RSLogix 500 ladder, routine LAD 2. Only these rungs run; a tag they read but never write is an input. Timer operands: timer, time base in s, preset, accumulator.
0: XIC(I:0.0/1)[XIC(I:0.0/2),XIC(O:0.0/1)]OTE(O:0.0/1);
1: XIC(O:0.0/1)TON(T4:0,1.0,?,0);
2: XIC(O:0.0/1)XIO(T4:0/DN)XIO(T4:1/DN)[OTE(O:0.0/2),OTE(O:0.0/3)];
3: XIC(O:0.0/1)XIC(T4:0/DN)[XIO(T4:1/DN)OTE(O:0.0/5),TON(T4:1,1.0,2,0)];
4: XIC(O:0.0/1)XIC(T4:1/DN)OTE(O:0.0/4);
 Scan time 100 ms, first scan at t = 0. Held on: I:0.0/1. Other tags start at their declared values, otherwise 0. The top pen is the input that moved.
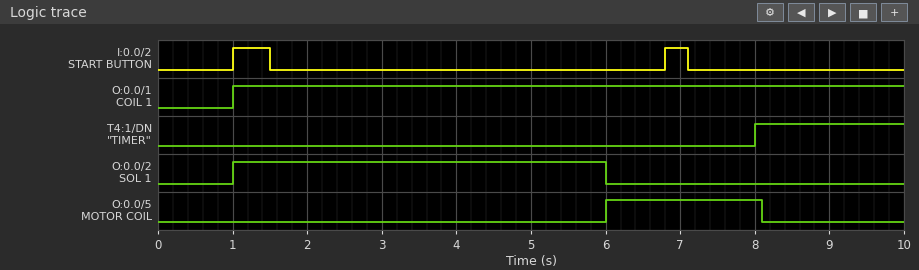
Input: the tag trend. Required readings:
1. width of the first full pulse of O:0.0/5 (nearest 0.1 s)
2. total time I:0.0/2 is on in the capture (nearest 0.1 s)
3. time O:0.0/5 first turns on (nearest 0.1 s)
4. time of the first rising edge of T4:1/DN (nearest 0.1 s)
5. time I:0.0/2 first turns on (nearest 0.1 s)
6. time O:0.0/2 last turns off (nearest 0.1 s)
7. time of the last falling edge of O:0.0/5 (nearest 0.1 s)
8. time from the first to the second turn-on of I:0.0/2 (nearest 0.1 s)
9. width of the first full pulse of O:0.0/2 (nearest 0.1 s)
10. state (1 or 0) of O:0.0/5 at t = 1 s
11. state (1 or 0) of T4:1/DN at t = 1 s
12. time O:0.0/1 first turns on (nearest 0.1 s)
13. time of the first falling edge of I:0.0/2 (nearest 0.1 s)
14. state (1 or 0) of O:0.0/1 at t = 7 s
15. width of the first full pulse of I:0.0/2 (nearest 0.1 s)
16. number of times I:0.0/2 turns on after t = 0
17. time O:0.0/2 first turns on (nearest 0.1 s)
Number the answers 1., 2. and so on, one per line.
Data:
1. 2.1 s
2. 0.8 s
3. 6.0 s
4. 8.0 s
5. 1.0 s
6. 6.0 s
7. 8.1 s
8. 5.8 s
9. 5.0 s
10. 0
11. 0
12. 1.0 s
13. 1.5 s
14. 1
15. 0.5 s
16. 2
17. 1.0 s
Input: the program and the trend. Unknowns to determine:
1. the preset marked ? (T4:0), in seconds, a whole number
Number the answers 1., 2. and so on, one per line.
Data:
1. 5 s
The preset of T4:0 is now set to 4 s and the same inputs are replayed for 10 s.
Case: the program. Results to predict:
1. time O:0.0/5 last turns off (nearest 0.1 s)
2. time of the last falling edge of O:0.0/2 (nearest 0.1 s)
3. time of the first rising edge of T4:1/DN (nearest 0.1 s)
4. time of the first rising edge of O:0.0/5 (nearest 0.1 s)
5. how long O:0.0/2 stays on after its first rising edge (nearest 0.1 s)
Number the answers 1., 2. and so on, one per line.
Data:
1. 7.1 s
2. 5.0 s
3. 7.0 s
4. 5.0 s
5. 4.0 s
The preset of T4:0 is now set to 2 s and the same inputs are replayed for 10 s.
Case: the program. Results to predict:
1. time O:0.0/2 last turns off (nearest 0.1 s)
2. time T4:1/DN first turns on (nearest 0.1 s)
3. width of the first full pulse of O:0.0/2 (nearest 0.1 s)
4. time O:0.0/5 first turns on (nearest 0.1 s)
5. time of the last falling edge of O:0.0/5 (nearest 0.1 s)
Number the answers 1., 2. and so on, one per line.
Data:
1. 3.0 s
2. 5.0 s
3. 2.0 s
4. 3.0 s
5. 5.1 s
